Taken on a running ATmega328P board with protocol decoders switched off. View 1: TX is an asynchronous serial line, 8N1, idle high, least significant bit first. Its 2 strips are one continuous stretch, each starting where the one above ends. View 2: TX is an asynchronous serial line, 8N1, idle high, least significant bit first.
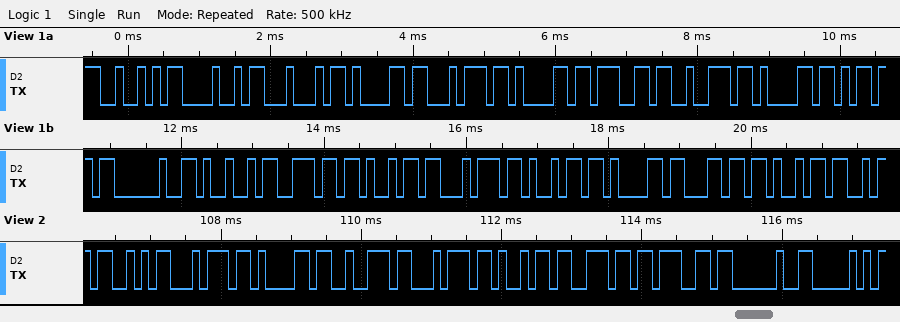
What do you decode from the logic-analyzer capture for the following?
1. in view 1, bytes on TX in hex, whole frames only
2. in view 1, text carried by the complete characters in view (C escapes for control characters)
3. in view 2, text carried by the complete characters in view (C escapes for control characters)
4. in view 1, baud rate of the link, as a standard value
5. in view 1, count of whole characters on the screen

0x52 0x48 0x44 0x61 0x74 0x61 0x67 0x72 0x61 0x6D 0x20 0x49 0x6E 0x69 0x74 0x69 0x61 0x6C 0x69
"RHDatagram Initiali"
"Starting P"
9600 baud
19
